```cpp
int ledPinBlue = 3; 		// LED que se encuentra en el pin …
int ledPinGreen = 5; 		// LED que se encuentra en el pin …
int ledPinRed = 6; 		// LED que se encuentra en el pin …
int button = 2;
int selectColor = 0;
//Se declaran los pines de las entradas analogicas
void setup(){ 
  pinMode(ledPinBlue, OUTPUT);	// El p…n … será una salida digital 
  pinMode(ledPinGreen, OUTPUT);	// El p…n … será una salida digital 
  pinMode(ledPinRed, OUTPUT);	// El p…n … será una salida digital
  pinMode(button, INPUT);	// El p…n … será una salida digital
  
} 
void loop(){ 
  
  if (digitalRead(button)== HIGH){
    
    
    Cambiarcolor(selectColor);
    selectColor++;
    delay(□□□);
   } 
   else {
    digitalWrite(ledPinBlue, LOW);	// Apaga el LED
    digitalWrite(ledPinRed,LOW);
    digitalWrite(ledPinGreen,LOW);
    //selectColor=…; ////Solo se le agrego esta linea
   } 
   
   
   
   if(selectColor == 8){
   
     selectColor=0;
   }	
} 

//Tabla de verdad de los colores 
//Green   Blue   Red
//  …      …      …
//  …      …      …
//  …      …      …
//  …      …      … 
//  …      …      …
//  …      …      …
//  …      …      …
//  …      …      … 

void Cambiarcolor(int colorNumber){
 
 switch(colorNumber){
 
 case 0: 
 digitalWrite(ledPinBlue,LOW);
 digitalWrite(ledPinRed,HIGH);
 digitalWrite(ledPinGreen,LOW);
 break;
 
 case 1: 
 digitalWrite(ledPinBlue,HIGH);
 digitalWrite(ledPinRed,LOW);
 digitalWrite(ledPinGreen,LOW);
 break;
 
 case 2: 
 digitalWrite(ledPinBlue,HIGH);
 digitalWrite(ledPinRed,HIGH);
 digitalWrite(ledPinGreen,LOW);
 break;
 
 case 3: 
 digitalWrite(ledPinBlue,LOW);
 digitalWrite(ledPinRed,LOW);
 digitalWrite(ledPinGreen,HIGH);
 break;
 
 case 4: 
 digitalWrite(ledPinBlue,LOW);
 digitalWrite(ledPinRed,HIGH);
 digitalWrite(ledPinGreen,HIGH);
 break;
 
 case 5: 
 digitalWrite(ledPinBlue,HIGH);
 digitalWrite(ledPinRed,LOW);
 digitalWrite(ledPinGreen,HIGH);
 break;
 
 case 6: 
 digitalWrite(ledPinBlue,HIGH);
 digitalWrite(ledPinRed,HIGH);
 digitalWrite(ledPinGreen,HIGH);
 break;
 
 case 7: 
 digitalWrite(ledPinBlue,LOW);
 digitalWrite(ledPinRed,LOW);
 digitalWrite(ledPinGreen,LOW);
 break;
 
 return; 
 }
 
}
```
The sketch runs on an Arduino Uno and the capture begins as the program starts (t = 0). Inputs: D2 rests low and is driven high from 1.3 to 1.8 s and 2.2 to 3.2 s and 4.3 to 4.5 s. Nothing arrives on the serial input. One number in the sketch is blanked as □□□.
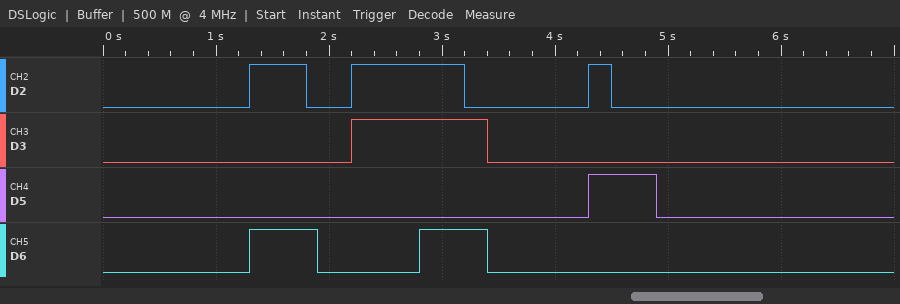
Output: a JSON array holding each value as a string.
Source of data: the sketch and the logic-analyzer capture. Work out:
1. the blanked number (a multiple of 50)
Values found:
["600"]
